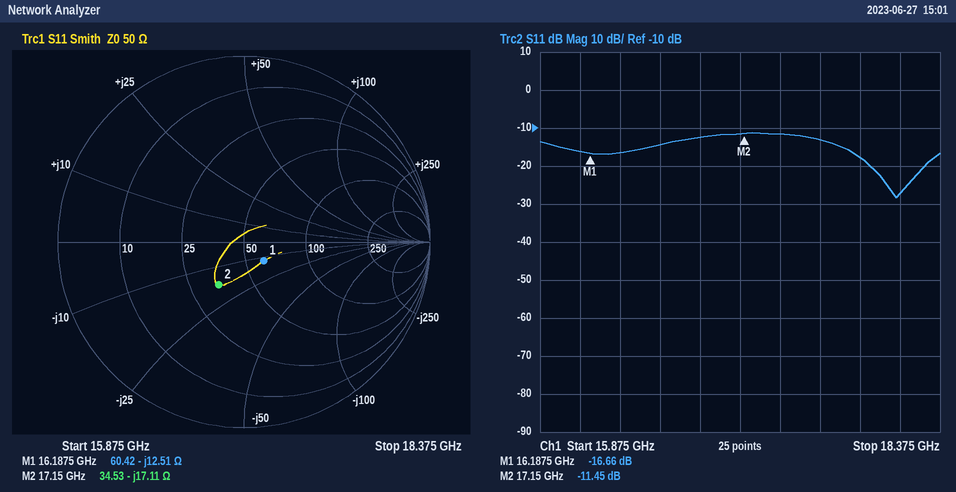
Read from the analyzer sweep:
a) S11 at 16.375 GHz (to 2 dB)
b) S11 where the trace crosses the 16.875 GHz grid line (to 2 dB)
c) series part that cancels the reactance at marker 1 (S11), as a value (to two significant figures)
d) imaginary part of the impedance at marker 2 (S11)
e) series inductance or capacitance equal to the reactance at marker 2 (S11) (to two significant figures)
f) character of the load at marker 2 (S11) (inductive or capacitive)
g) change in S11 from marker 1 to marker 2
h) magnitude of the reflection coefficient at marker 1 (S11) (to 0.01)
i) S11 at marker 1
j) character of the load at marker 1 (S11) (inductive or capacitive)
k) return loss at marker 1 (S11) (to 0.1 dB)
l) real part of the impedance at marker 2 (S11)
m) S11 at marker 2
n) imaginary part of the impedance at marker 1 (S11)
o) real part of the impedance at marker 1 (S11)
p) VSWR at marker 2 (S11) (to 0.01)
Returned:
-16 dB
-12 dB
120 pH
-17.11 Ω
540 fF
capacitive
5.21 dB
0.15
-16.66 dB
capacitive
16.7 dB
34.53 Ω
-11.45 dB
-12.51 Ω
60.42 Ω
1.73
